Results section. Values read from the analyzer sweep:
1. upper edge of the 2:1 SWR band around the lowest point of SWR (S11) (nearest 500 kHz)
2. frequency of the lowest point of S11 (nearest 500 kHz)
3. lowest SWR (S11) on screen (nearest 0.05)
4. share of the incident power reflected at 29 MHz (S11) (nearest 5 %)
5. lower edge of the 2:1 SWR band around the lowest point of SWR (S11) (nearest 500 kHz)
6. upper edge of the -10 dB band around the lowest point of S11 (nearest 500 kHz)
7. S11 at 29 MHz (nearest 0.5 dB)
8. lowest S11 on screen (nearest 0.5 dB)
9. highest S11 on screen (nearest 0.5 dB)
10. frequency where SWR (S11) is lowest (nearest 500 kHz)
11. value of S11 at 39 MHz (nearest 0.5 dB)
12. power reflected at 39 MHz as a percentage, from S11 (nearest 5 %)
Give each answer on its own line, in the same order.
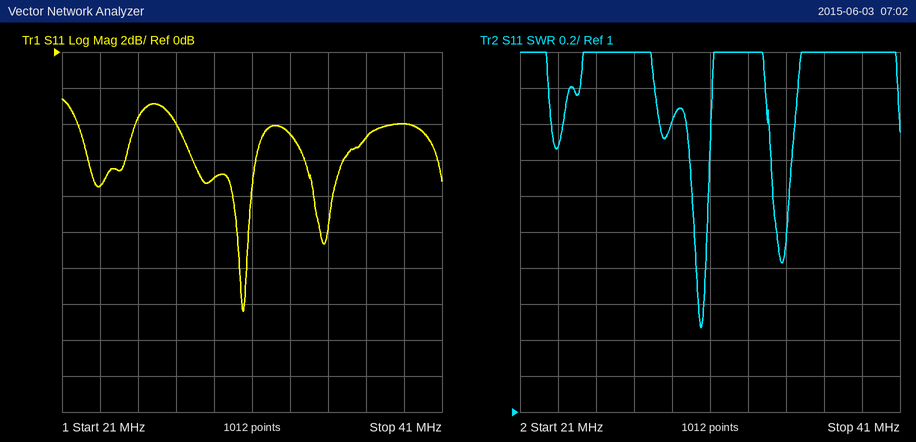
31.0 MHz
30.5 MHz
1.45
20 %
30.0 MHz
31.0 MHz
-7.0 dB
-14.5 dB
-2.5 dB
30.5 MHz
-4.0 dB
40 %
